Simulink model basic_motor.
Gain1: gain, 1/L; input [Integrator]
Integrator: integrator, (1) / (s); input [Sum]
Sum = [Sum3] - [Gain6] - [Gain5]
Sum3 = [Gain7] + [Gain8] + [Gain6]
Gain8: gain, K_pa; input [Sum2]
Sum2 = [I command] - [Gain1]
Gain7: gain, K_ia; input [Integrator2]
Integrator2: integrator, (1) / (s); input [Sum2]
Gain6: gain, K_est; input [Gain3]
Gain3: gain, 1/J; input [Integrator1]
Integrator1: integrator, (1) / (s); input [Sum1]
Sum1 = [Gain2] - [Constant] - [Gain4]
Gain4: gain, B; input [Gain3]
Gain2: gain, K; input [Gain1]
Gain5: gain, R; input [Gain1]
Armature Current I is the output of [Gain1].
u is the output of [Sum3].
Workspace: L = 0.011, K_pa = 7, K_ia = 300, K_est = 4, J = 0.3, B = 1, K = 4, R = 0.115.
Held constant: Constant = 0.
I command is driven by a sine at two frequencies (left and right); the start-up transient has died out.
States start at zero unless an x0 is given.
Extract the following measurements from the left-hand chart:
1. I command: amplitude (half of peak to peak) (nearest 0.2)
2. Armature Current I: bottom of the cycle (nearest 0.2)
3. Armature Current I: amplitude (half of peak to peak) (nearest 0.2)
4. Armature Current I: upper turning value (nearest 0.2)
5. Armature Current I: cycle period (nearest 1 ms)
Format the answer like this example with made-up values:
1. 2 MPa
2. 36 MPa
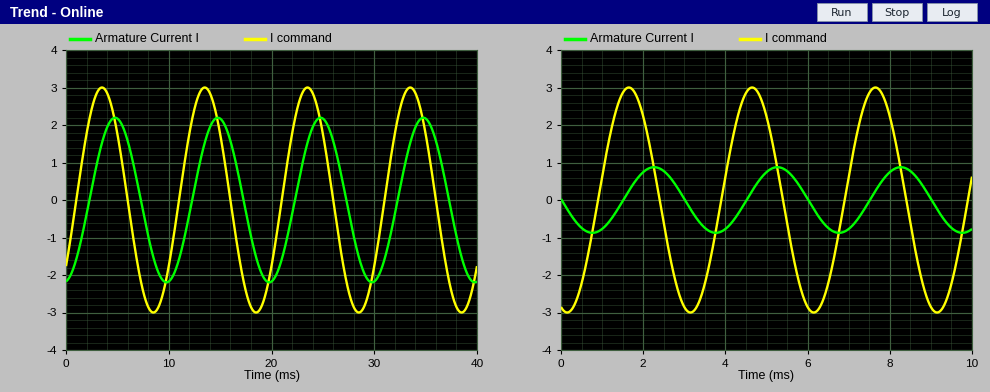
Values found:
1. 3.0
2. -2.2
3. 2.2
4. 2.2
5. 10 ms
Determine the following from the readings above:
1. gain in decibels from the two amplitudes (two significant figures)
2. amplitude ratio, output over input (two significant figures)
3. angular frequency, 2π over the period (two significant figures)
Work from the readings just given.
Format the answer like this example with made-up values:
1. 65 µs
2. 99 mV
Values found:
1. -2.7 dB
2. 0.73
3. 0.63 rad/ms
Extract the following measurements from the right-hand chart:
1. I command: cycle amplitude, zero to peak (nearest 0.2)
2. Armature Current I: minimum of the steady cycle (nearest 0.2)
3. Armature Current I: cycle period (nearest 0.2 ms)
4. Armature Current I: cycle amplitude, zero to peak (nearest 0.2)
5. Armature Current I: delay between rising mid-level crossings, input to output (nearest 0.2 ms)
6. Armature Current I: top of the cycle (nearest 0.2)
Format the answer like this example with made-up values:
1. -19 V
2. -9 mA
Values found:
1. 3.0
2. -0.8
3. 3.0 ms
4. 0.8
5. 0.6 ms
6. 0.8
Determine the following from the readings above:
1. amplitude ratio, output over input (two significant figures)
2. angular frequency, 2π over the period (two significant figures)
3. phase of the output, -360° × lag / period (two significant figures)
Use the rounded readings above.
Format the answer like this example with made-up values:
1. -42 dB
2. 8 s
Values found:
1. 0.27
2. 2.1 rad/ms
3. -72°
